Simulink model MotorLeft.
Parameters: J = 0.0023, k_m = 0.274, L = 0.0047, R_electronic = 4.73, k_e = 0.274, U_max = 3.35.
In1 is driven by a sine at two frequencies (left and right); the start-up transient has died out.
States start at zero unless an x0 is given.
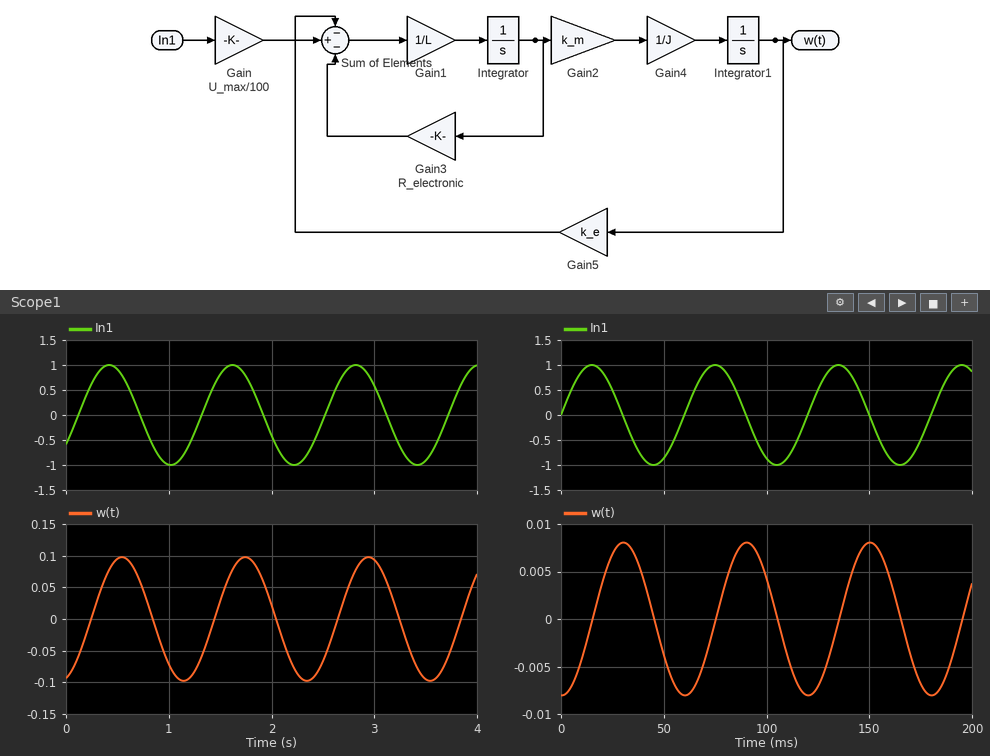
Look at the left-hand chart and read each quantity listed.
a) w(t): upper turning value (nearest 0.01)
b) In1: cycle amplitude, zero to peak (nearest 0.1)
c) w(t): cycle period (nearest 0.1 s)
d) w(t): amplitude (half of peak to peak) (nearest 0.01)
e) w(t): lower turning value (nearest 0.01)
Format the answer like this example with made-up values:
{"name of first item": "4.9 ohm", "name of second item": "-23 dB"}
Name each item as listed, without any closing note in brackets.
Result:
{"w(t): upper turning value": "0.10", "In1: cycle amplitude, zero to peak": "1.0", "w(t): cycle period": "1.2 s", "w(t): amplitude (half of peak to peak)": "0.10", "w(t): lower turning value": "-0.10"}
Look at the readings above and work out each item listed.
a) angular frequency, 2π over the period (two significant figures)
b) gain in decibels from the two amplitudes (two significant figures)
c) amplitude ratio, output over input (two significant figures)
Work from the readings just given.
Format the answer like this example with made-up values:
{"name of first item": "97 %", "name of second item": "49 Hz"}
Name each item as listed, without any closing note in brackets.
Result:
{"angular frequency, 2π over the period": "5.2 rad/s", "gain in decibels from the two amplitudes": "-20 dB", "amplitude ratio, output over input": "0.10"}
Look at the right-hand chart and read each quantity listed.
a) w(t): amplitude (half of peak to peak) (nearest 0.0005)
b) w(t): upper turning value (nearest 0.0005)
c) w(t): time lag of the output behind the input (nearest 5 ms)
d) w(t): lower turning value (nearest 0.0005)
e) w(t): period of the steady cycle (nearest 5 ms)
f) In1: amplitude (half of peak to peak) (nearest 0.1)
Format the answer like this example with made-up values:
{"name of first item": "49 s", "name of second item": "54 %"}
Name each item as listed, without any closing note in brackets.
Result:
{"w(t): amplitude (half of peak to peak)": "0.0080", "w(t): upper turning value": "0.0080", "w(t): time lag of the output behind the input": "15 ms", "w(t): lower turning value": "-0.0080", "w(t): period of the steady cycle": "60 ms", "In1: amplitude (half of peak to peak)": "1.0"}
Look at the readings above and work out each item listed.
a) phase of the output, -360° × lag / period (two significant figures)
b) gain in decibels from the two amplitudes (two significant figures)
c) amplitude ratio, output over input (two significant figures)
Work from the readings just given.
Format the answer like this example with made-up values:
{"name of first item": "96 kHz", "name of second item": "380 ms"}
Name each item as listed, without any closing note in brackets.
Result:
{"phase of the output, -360° × lag / period": "-90°", "gain in decibels from the two amplitudes": "-42 dB", "amplitude ratio, output over input": "0.0080"}
